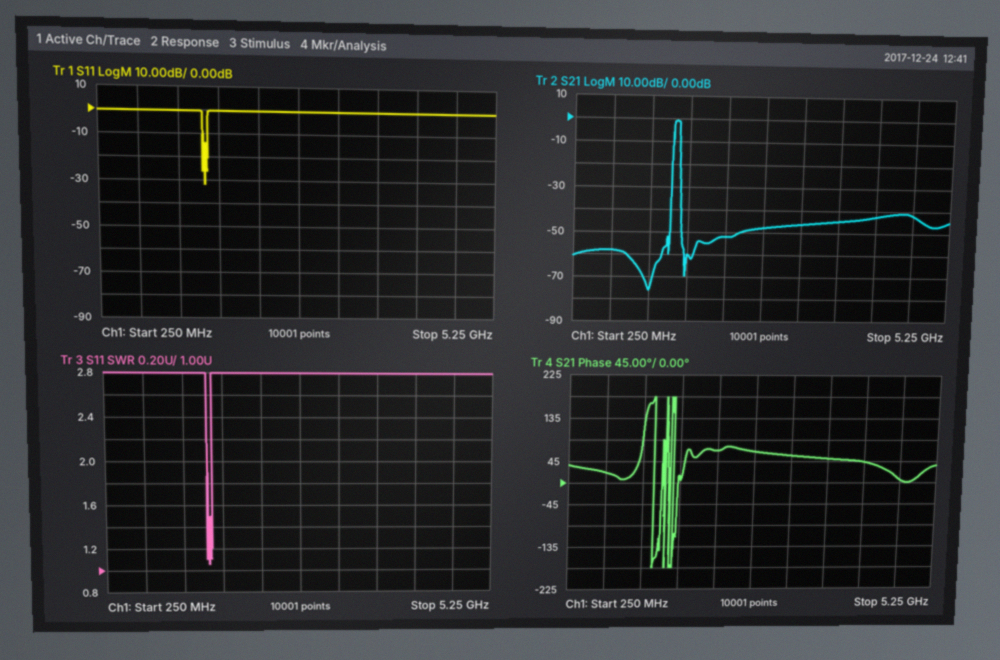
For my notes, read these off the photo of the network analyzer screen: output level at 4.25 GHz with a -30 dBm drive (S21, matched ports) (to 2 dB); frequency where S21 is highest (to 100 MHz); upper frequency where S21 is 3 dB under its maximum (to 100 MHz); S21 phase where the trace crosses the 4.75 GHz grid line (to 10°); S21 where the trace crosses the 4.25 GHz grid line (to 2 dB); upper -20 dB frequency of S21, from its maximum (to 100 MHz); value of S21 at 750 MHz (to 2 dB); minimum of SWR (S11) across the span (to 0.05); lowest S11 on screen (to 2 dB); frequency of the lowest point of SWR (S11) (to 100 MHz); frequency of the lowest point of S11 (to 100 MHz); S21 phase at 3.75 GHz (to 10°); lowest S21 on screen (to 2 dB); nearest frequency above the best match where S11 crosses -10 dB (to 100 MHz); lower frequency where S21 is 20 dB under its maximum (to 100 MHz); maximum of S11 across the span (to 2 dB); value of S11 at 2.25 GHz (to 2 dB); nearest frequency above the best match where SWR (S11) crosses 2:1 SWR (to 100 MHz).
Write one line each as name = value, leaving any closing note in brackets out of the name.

output level at 4.25 GHz with a -30 dBm drive (S21, matched ports) = -72 dBm
frequency where S21 is highest = 1.6 GHz
upper frequency where S21 is 3 dB under its maximum = 1.6 GHz
S21 phase where the trace crosses the 4.75 GHz grid line = 10°
S21 where the trace crosses the 4.25 GHz grid line = -42 dB
upper -20 dB frequency of S21, from its maximum = 1.6 GHz
value of S21 at 750 MHz = -58 dB
minimum of SWR (S11) across the span = 1.05
lowest S11 on screen = -32 dB
frequency of the lowest point of SWR (S11) = 1.6 GHz
frequency of the lowest point of S11 = 1.6 GHz
S21 phase at 3.75 GHz = 50°
lowest S21 on screen = -76 dB
nearest frequency above the best match where S11 crosses -10 dB = 1.6 GHz
lower frequency where S21 is 20 dB under its maximum = 1.5 GHz
maximum of S11 across the span = 0 dB
value of S11 at 2.25 GHz = 0 dB
nearest frequency above the best match where SWR (S11) crosses 2:1 SWR = 1.6 GHz
